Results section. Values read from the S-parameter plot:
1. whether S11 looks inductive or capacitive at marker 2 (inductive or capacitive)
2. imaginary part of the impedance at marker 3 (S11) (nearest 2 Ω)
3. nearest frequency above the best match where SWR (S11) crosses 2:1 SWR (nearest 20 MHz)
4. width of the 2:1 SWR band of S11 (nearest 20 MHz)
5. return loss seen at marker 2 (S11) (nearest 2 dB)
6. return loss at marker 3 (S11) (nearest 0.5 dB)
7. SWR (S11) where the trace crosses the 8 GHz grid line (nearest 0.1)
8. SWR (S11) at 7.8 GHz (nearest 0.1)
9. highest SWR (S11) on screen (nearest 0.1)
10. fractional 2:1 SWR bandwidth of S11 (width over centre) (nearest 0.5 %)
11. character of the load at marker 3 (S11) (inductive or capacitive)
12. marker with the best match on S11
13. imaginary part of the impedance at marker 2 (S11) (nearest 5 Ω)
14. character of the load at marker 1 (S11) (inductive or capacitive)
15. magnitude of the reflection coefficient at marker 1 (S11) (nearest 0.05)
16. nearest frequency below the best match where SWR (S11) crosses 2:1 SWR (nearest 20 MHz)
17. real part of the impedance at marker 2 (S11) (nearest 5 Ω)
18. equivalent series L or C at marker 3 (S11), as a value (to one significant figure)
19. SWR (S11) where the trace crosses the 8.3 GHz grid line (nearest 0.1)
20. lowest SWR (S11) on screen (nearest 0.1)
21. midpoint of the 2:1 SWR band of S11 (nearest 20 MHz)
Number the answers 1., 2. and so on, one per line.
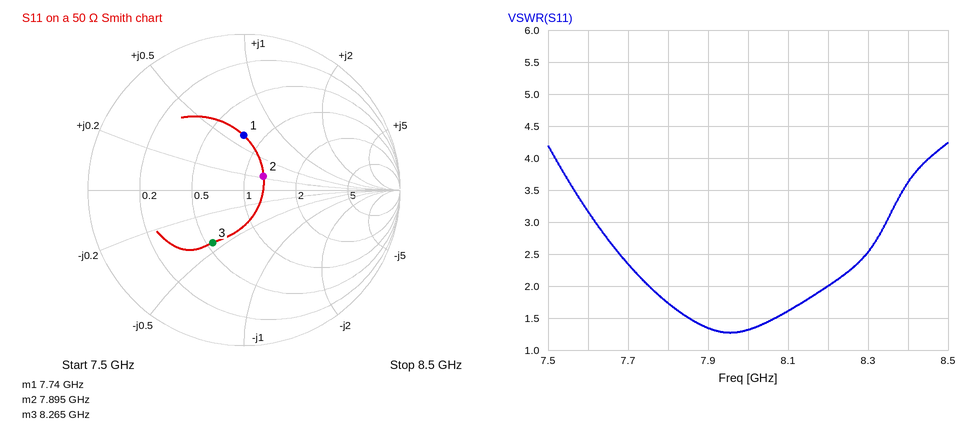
1. inductive
2. -22 Ω
3. 8.20 GHz
4. 440 MHz
5. 16 dB
6. 8.0 dB
7. 1.3
8. 1.7
9. 4.2
10. 5.5 %
11. capacitive
12. marker 2
13. +10 Ω
14. inductive
15. 0.35
16. 7.76 GHz
17. 65 Ω
18. 900 fF
19. 2.5
20. 1.3
21. 7.98 GHz
